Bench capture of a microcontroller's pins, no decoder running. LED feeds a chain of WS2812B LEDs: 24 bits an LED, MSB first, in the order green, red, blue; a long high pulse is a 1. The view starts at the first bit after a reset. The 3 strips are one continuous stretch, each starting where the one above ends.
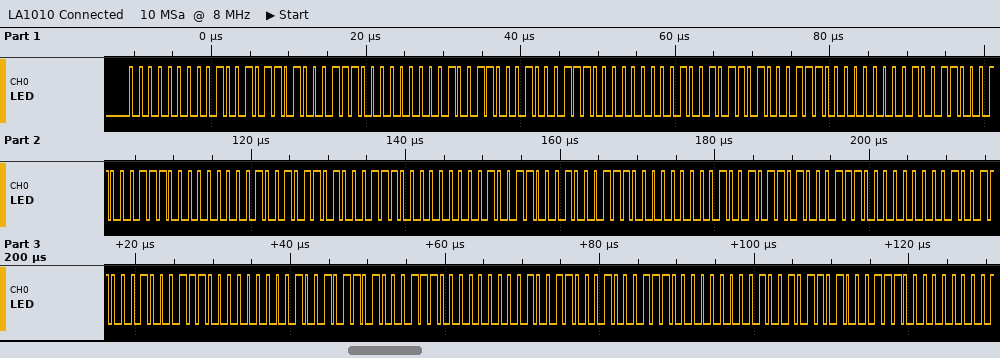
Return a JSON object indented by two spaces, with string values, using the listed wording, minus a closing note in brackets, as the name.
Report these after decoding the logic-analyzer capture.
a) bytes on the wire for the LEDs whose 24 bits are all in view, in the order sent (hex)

{
  "bytes on the wire for the LEDs whose 24 bits are all in view, in the order sent": "00 4B 47 00 4C 47 00 4B 47 00 4C 47 00 4B 47 00 4C 47 00 4B 47 00 4C 47 00 4B 47 00 4C 47 00 4B 47"
}
